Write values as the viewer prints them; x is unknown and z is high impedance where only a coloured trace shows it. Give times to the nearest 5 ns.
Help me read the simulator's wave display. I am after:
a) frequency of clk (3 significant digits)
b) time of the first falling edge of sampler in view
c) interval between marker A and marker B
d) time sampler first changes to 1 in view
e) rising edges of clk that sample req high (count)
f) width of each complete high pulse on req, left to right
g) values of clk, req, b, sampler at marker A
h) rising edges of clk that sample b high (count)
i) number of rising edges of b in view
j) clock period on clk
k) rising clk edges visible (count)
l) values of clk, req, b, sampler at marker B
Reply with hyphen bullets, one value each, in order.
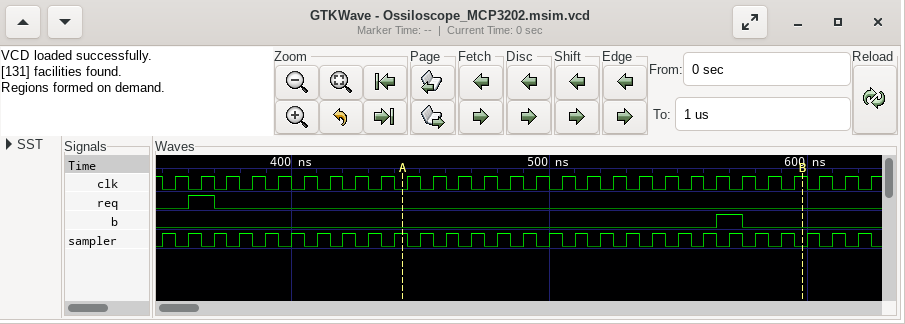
- 100 MHz
- 355 ns
- 155 ns
- 350 ns
- 1
- 10 ns
- clk=0, req=0, b=0, sampler=1
- 1
- 1
- 10 ns
- 28
- clk=1, req=0, b=0, sampler=0
